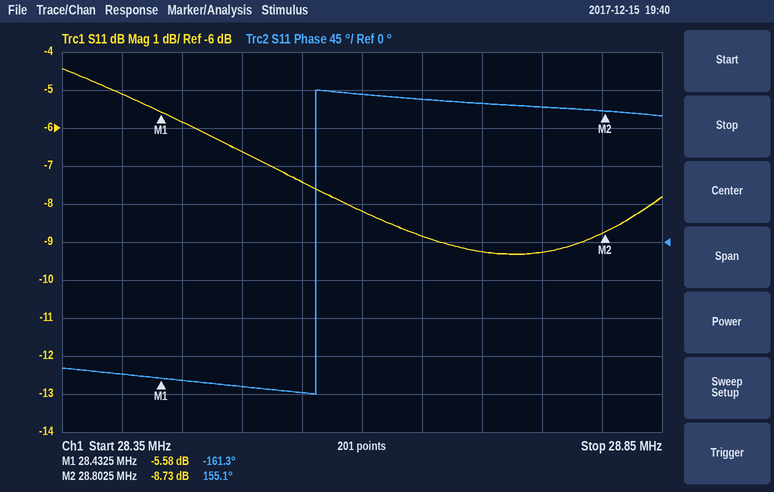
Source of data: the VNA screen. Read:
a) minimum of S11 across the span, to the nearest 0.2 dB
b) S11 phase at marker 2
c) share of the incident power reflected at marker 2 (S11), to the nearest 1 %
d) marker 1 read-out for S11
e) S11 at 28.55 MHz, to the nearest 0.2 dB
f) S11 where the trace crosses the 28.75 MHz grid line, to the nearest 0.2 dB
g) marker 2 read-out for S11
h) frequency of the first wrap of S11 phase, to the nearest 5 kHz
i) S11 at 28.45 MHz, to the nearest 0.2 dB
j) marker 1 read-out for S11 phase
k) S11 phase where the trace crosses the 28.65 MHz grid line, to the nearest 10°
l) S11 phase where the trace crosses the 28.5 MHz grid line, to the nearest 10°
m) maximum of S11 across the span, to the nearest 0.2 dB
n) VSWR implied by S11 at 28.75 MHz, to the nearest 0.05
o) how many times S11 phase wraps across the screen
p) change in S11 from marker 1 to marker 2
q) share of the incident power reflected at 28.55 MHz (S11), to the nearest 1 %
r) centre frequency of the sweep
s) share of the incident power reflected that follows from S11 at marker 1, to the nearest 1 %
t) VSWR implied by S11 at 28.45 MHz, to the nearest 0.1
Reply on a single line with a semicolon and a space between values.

-9.4 dB; 155.1°; 13 %; -5.58 dB; -7.4 dB; -9.2 dB; -8.73 dB; 28.560 MHz; -5.8 dB; -161.3°; 170°; -170°; -4.4 dB; 2.05; 1; -3.15 dB; 18 %; 28.6 MHz; 28 %; 3.1
